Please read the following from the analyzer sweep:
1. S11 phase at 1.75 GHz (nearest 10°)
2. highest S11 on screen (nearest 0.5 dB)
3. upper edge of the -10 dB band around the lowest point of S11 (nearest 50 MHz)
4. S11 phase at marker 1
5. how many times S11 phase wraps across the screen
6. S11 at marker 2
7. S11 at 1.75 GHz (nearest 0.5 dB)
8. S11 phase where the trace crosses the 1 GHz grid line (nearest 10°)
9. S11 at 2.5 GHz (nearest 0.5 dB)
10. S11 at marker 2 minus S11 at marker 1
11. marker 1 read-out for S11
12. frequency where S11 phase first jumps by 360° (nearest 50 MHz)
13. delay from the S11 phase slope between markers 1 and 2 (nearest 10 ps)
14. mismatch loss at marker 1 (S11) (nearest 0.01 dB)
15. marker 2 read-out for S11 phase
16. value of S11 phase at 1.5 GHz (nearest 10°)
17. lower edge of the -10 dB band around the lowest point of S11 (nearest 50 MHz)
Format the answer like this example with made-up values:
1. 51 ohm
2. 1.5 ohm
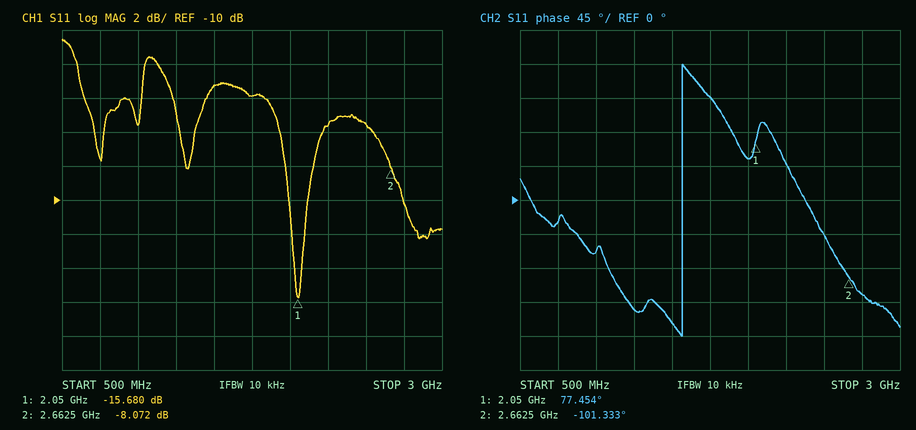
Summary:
1. 140°
2. -0.5 dB
3. 2.10 GHz
4. 77.454°
5. 1
6. -8.072 dB
7. -4.0 dB
8. -70°
9. -5.5 dB
10. 7.608 dB
11. -15.680 dB
12. 1.55 GHz
13. 810 ps
14. 0.12 dB
15. -101.333°
16. -160°
17. 2.00 GHz
